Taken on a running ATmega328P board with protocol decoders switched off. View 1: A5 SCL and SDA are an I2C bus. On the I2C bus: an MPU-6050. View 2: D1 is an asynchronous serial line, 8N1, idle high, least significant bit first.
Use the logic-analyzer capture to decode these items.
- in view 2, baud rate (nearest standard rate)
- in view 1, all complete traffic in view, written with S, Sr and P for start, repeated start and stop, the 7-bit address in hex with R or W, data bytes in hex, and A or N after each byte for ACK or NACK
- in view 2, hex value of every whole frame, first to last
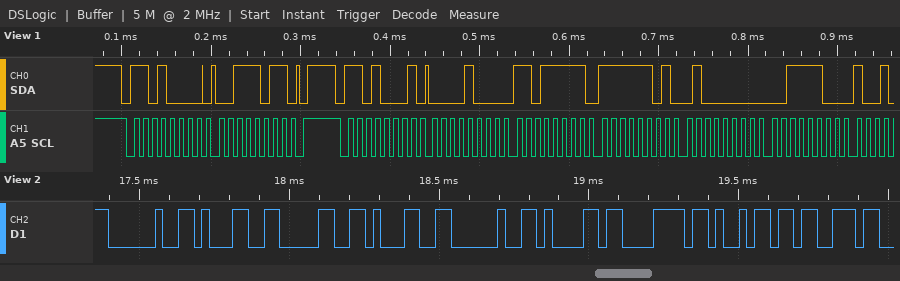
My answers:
38400 baud
S 68W A 3B A P S 68R A 08 A DF A FD A 40 A 3C A
20 31 30 31 20 61 78 69 73
